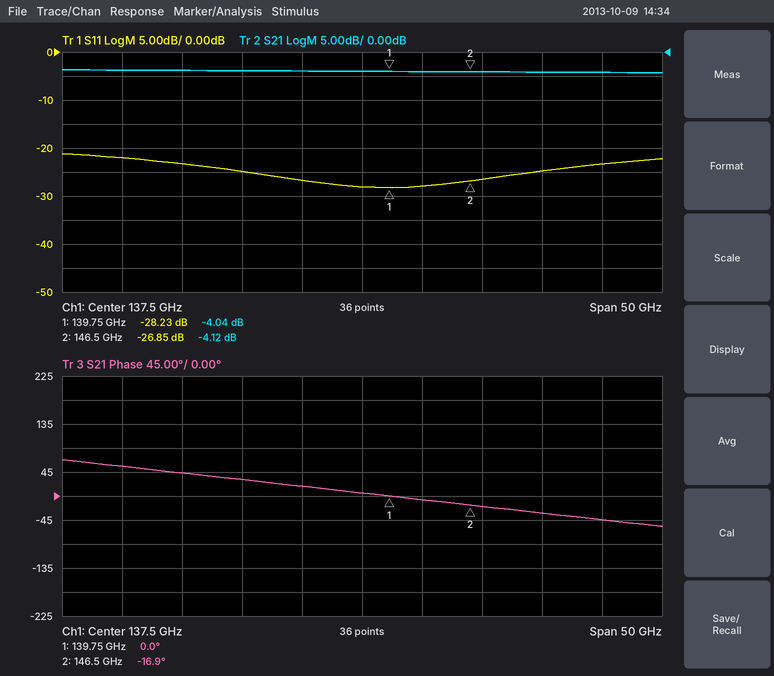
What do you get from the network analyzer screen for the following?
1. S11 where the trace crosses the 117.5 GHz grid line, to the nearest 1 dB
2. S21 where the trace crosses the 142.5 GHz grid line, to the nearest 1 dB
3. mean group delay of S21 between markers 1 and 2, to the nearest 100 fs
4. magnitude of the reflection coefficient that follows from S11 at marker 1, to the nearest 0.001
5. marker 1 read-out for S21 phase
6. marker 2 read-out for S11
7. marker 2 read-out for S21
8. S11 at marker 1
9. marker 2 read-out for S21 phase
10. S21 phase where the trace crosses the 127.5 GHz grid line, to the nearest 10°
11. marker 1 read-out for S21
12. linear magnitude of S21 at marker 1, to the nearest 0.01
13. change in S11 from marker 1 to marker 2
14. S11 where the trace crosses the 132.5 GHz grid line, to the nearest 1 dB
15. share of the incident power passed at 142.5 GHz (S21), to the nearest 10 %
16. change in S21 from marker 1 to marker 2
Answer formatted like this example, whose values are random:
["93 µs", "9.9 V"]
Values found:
["-22 dB", "-4 dB", "7.0 ps", "0.039", "0.0°", "-26.85 dB", "-4.12 dB", "-28.23 dB", "-16.9°", "30°", "-4.04 dB", "0.63", "1.38 dB", "-27 dB", "40 %", "-0.08 dB"]
